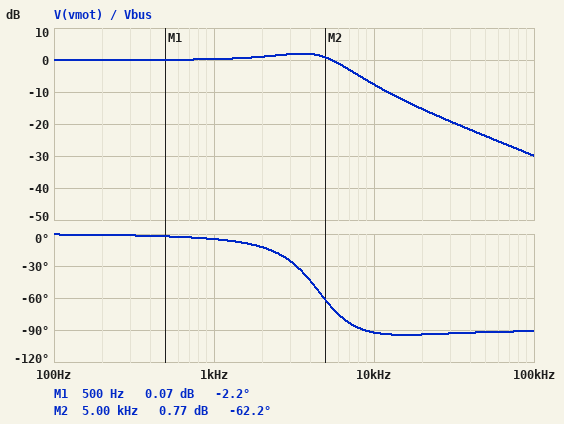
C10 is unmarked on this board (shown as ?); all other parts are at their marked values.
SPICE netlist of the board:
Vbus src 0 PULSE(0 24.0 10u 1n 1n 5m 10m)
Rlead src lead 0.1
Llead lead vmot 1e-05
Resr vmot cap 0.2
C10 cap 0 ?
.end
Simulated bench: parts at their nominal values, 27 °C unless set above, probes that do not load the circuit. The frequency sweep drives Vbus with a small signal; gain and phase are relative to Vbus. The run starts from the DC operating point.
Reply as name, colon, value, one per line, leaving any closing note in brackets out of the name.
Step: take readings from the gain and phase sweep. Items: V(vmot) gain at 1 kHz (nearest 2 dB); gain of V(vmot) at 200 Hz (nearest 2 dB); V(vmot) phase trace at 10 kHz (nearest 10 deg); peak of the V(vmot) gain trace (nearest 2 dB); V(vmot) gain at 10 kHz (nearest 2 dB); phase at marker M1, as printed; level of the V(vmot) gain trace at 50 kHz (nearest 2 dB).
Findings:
V(vmot) gain at 1 kHz: 0 dB
gain of V(vmot) at 200 Hz: 0 dB
V(vmot) phase trace at 10 kHz: -90 deg
peak of the V(vmot) gain trace: 2 dB
V(vmot) gain at 10 kHz: -8 dB
phase at marker M1, as printed: -2.2 deg
level of the V(vmot) gain trace at 50 kHz: -24 dB
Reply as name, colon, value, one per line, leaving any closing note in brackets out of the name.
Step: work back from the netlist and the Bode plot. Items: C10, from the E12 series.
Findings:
C10, from the E12 series: 120 µF
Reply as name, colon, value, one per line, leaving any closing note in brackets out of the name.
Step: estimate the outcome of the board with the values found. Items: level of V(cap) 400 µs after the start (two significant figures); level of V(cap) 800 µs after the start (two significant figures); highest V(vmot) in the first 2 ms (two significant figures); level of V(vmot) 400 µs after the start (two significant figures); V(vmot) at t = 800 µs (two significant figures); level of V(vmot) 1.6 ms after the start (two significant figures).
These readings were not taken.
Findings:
level of V(cap) 400 µs after the start: 24 V
level of V(cap) 800 µs after the start: 24 V
highest V(vmot) in the first 2 ms: 29 V
level of V(vmot) 400 µs after the start: 24 V
V(vmot) at t = 800 µs: 24 V
level of V(vmot) 1.6 ms after the start: 24 V
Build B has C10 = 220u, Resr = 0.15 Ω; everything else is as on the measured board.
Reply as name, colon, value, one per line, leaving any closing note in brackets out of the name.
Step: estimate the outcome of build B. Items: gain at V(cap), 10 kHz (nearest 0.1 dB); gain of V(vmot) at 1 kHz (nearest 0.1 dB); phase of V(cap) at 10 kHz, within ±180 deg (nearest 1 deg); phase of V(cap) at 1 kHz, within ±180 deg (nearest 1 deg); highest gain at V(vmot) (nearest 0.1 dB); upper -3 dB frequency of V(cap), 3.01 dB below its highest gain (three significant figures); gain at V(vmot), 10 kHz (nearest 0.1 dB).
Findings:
gain at V(cap), 10 kHz: -18.5 dB
gain of V(vmot) at 1 kHz: 0.4 dB
phase of V(cap) at 10 kHz, within ±180 deg: -156 deg
phase of V(cap) at 1 kHz, within ±180 deg: -21 deg
highest gain at V(vmot): 1.2 dB
upper -3 dB frequency of V(cap), 3.01 dB below its highest gain: 3.81 kHz
gain at V(vmot), 10 kHz: -11.3 dB
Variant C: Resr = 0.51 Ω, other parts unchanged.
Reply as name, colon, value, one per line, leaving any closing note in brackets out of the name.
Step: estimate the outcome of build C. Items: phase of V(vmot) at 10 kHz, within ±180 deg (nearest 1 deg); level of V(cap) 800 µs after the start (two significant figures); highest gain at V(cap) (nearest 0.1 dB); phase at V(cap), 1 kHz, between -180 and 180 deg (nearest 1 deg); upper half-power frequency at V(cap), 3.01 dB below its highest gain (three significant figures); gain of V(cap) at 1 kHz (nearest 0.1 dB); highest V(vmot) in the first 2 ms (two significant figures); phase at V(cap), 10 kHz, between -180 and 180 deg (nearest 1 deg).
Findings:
phase of V(vmot) at 10 kHz, within ±180 deg: -54 deg
level of V(cap) 800 µs after the start: 24 V
highest gain at V(cap): 0 dB
phase at V(cap), 1 kHz, between -180 and 180 deg: -26 deg
upper half-power frequency at V(cap), 3.01 dB below its highest gain: 2.74 kHz
gain of V(cap) at 1 kHz: -0.5 dB
highest V(vmot) in the first 2 ms: 25 V
phase at V(cap), 10 kHz, between -180 and 180 deg: -129 deg
